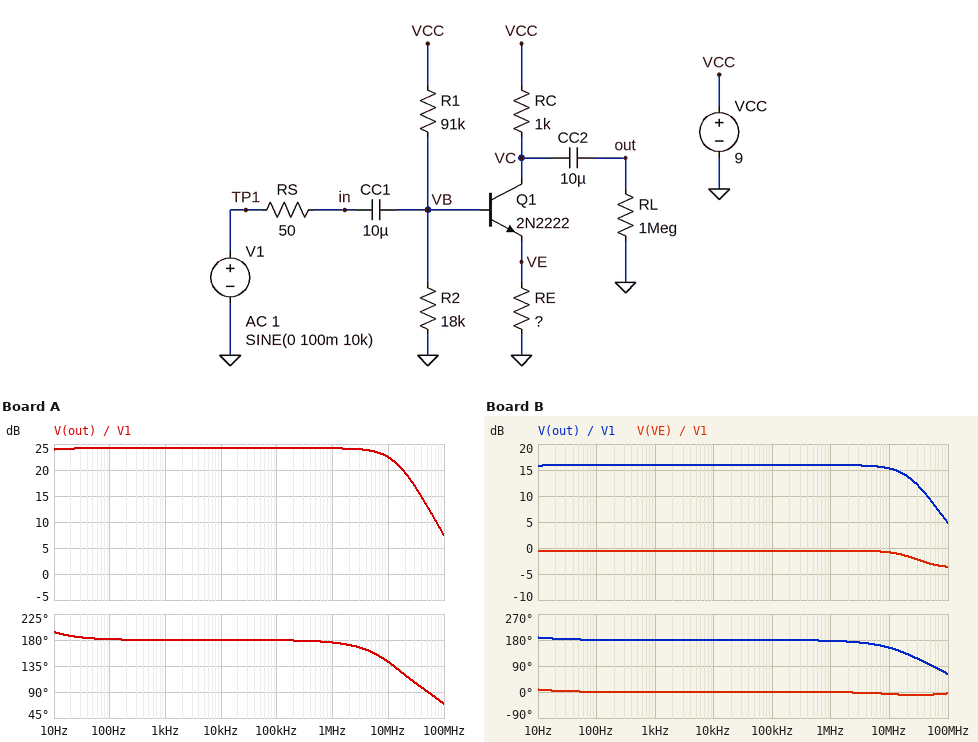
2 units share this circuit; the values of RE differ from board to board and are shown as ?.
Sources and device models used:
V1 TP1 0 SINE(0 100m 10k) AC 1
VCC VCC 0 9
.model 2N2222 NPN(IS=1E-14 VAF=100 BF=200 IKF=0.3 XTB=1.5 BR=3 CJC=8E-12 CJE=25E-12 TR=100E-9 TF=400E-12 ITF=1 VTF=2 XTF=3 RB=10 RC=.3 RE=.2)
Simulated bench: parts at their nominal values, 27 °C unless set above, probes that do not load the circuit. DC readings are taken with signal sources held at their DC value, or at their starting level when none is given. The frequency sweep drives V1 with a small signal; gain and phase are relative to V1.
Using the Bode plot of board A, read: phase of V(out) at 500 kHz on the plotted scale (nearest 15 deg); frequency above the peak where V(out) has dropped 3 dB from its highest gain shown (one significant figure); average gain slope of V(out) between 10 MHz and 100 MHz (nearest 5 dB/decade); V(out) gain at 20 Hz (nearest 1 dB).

180 deg
10 MHz
-15 dB/decade
24 dB
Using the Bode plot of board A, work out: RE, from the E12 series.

56 Ω
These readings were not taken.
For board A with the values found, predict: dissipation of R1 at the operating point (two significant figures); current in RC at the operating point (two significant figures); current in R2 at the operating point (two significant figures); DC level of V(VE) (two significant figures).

700 µW
6.0 mA
58 µA
340 mV
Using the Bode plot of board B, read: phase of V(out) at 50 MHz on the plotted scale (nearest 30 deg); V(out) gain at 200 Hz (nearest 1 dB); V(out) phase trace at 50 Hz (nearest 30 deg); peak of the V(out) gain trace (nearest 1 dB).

90 deg
16 dB
180 deg
16 dB
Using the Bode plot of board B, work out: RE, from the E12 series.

150 Ω
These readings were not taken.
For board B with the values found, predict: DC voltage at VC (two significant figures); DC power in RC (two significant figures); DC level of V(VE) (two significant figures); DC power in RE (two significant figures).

5.4 V
13 mW
540 mV
1.9 mW
